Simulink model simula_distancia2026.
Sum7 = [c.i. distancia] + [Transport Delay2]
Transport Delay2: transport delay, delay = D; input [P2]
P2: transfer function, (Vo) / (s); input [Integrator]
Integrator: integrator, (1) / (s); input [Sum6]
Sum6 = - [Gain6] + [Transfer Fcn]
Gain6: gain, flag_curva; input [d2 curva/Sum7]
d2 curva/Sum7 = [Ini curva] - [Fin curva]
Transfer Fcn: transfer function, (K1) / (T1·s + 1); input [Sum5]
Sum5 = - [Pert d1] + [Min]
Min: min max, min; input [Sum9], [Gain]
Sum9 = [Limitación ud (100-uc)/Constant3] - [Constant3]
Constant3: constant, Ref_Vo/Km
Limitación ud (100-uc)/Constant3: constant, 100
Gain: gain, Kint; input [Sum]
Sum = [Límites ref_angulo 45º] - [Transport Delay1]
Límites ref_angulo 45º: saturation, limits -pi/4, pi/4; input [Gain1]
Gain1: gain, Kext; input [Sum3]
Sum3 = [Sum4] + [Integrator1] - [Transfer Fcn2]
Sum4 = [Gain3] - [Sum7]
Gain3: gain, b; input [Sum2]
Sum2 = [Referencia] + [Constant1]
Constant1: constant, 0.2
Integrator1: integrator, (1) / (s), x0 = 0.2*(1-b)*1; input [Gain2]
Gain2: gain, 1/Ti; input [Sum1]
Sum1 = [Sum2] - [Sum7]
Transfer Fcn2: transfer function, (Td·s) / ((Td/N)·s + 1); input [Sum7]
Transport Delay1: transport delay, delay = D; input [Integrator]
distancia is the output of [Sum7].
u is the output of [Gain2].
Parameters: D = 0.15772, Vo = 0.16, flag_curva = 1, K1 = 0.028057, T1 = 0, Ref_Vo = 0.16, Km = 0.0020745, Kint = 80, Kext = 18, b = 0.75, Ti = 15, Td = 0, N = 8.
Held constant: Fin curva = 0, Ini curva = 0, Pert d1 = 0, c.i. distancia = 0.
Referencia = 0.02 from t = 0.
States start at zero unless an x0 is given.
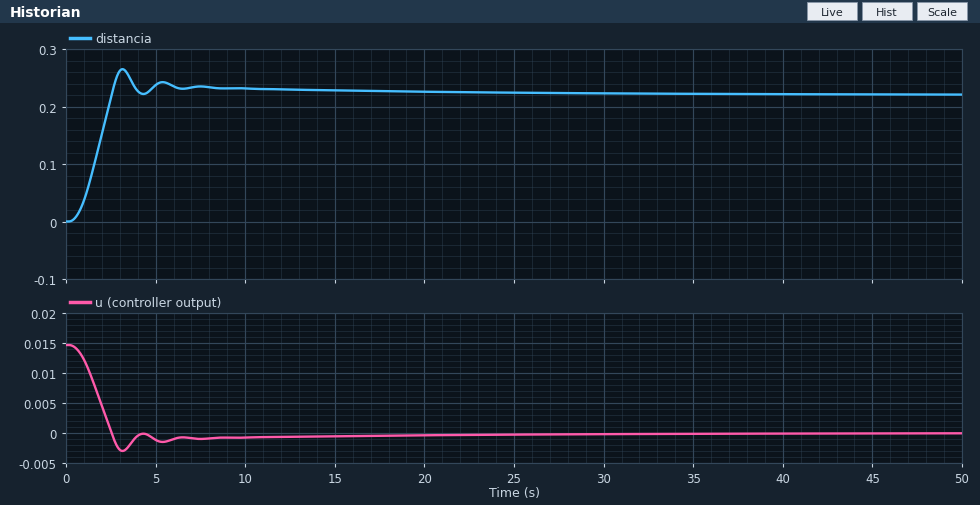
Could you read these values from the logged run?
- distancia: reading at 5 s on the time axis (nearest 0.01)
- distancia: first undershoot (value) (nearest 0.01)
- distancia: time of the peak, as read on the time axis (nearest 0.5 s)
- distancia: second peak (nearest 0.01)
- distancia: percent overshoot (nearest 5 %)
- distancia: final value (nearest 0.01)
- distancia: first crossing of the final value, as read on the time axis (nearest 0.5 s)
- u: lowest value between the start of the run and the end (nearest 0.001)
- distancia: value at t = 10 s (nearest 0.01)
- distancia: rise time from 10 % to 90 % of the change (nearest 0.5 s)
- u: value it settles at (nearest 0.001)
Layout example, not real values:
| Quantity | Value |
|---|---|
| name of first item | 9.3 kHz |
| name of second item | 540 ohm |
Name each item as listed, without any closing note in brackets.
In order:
| Quantity | Value |
|---|---|
| distancia: reading at 5 s on the time axis | 0.24 |
| distancia: first undershoot (value) | 0.22 |
| distancia: time of the peak, as read on the time axis | 3.0 s |
| distancia: second peak | 0.24 |
| distancia: percent overshoot | 20 % |
| distancia: final value | 0.22 |
| distancia: first crossing of the final value, as read on the time axis | 2.5 s |
| u: lowest value between the start of the run and the end | -0.003 |
| distancia: value at t = 10 s | 0.23 |
| distancia: rise time from 10 % to 90 % of the change | 1.5 s |
| u: value it settles at | 0.000 |
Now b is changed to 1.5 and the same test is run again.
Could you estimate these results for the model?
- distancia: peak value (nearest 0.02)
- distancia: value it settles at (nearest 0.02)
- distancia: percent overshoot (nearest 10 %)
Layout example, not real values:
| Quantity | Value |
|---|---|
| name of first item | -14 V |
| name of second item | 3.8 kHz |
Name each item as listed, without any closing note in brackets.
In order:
| Quantity | Value |
|---|---|
| distancia: peak value | 0.28 |
| distancia: value it settles at | 0.22 |
| distancia: percent overshoot | 30 % |
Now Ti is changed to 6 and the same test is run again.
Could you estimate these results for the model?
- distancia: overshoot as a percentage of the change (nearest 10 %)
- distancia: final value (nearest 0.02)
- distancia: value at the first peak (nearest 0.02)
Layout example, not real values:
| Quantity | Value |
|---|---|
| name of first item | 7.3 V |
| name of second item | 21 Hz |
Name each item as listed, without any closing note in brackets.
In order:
| Quantity | Value |
|---|---|
| distancia: overshoot as a percentage of the change | 40 % |
| distancia: final value | 0.22 |
| distancia: value at the first peak | 0.30 |
